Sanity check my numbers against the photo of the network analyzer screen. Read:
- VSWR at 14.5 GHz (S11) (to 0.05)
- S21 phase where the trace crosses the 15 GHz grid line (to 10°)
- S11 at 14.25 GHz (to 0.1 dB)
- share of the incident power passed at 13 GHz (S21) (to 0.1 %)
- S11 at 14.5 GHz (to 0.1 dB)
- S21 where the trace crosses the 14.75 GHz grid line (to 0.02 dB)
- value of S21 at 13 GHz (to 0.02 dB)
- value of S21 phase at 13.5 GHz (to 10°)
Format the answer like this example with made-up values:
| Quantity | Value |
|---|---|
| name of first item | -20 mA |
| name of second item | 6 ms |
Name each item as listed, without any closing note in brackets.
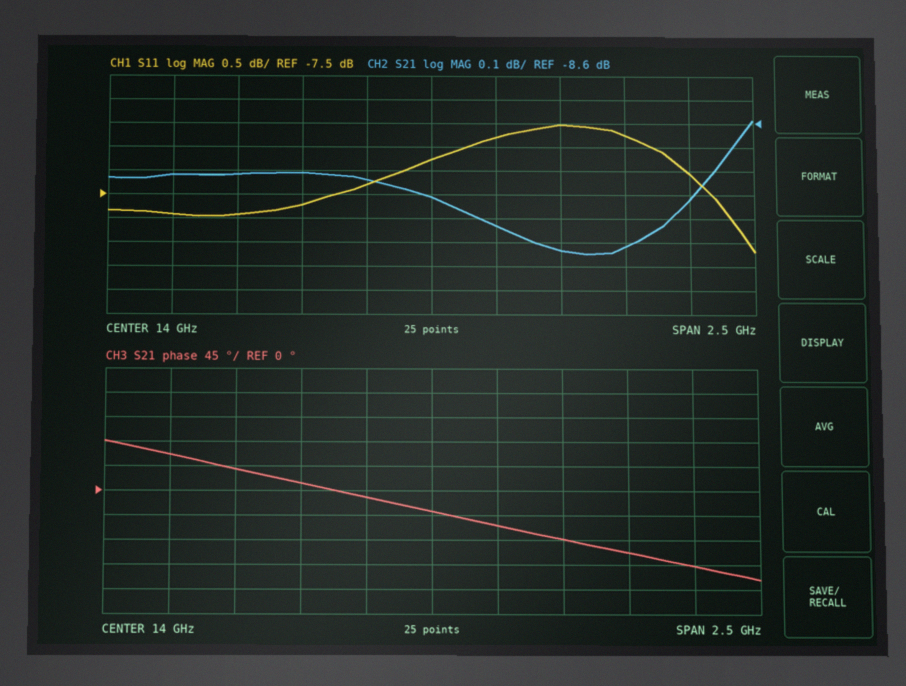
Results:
| Quantity | Value |
|---|---|
| VSWR at 14.5 GHz (S11) | 3.00 |
| S21 phase where the trace crosses the 15 GHz grid line | -140° |
| S11 at 14.25 GHz | -6.3 dB |
| share of the incident power passed at 13 GHz (S21) | 13.1 % |
| S11 at 14.5 GHz | -6.0 dB |
| S21 where the trace crosses the 14.75 GHz grid line | -9.12 dB |
| value of S21 at 13 GHz | -8.82 dB |
| value of S21 phase at 13.5 GHz | 10° |
